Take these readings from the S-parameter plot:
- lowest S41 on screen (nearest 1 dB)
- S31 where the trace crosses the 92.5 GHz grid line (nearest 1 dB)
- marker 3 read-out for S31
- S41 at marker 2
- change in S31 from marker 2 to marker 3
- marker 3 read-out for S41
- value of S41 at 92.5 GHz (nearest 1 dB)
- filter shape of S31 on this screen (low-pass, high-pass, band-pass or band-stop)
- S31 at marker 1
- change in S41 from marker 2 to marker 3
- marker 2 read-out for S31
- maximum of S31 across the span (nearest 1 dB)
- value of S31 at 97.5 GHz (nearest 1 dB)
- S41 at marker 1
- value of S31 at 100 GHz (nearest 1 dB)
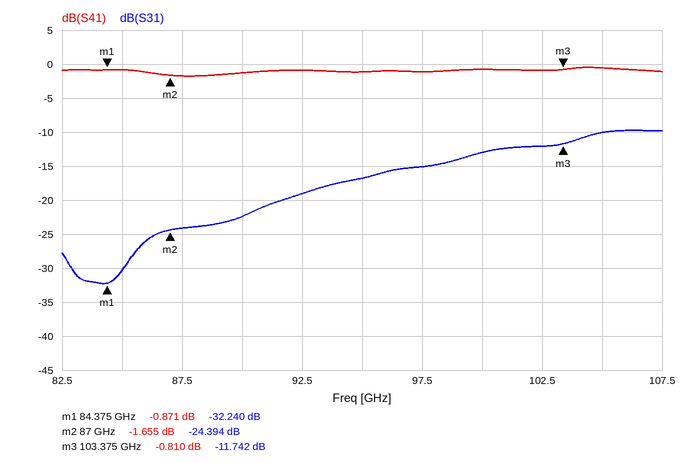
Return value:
-2 dB
-19 dB
-11.742 dB
-1.655 dB
12.652 dB
-0.810 dB
-1 dB
high-pass
-32.240 dB
0.845 dB
-24.394 dB
-10 dB
-15 dB
-0.871 dB
-13 dB
